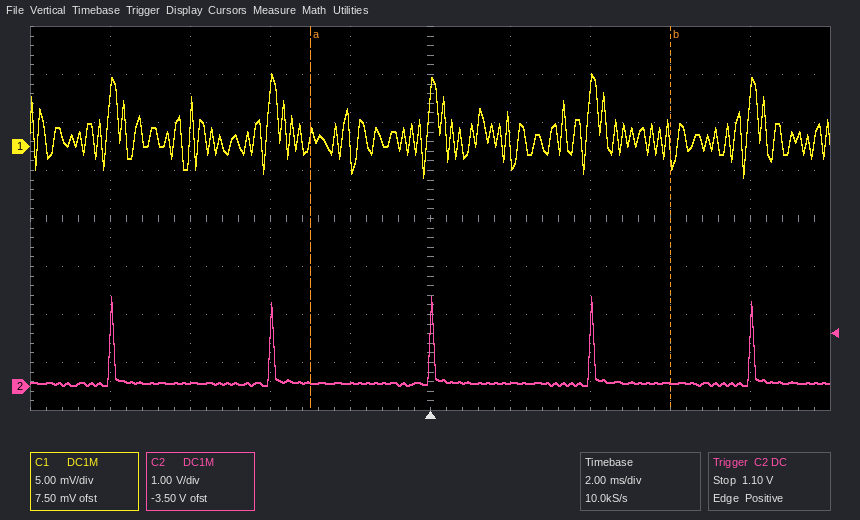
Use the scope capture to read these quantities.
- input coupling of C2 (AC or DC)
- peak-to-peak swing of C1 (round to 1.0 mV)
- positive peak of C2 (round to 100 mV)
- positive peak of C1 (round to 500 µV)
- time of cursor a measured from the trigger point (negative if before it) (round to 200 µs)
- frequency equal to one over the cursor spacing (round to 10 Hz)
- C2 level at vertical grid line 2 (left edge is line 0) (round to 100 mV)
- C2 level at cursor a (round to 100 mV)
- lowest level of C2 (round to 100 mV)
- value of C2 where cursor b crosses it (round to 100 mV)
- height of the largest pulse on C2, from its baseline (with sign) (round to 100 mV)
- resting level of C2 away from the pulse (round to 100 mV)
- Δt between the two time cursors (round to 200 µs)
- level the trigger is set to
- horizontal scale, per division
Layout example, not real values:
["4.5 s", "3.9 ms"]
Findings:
["DC", "11.0 mV", "1.9 V", "7.5 mV", "-3.0 ms", "110 Hz", "100 mV", "100 mV", "0.0 V", "100 mV", "+1.8 V", "100 mV", "9.0 ms", "1.10 V", "2 ms"]
